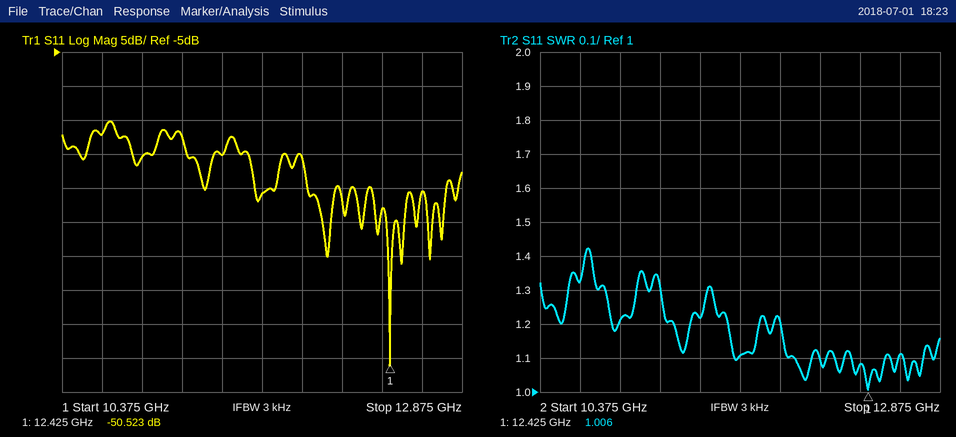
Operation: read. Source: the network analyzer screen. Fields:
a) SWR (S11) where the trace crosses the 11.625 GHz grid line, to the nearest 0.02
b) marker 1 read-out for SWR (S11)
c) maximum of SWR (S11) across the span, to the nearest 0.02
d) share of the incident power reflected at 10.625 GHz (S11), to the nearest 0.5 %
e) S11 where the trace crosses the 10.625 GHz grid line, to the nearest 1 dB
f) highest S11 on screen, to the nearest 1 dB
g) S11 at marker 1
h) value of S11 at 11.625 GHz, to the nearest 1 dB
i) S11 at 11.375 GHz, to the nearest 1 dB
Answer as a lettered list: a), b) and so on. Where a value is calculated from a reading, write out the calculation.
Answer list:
a) 1.10
b) 1.006
c) 1.42
d) 10^(-17/10) ≈ 2.0 %
e) -17 dB
f) -15 dB
g) -50.523 dB
h) -26 dB
i) -20 dB
